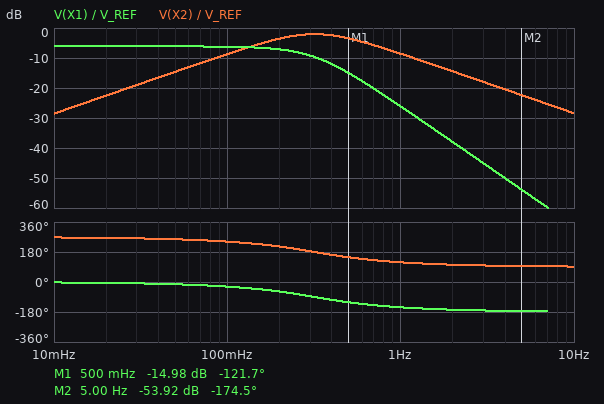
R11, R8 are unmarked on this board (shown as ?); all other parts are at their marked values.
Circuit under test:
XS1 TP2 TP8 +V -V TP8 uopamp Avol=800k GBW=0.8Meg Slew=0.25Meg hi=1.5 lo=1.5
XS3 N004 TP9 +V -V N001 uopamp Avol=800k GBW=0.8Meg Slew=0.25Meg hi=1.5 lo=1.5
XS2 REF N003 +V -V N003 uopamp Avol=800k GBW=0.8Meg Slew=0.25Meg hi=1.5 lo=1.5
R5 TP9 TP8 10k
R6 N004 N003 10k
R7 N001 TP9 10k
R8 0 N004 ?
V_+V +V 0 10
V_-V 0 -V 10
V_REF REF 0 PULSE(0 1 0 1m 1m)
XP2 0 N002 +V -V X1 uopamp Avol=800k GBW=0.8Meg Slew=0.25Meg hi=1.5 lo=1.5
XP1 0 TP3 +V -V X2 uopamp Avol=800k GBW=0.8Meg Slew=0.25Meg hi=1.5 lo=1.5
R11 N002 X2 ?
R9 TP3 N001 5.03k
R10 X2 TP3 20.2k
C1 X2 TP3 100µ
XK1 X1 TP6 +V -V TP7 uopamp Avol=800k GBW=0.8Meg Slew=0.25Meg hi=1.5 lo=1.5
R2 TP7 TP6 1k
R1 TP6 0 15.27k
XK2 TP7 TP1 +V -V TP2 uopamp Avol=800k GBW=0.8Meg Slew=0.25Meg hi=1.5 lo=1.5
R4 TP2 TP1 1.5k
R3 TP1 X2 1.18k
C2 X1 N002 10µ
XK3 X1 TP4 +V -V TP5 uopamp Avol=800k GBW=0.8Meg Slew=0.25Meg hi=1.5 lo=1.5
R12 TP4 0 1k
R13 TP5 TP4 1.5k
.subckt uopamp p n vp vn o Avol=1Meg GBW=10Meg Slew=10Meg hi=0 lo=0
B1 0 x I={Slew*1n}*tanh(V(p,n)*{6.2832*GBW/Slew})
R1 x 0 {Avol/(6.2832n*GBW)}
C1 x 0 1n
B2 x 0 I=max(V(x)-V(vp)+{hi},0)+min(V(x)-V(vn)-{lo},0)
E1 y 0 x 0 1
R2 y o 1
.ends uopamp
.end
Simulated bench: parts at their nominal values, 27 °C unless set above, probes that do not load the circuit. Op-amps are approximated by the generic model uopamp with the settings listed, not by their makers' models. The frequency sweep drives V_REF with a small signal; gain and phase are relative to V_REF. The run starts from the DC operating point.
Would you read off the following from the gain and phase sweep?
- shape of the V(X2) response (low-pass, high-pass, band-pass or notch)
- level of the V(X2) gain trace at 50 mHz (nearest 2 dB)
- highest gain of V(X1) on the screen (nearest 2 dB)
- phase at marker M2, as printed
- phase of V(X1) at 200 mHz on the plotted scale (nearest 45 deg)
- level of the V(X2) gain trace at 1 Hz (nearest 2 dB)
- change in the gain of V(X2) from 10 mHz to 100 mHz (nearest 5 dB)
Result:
band-pass
-14 dB
-6 dB
-174.5 deg
-45 deg
-8 dB
20 dB
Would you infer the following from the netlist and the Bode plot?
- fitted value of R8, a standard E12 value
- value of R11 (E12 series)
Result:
15 kΩ
120 kΩ
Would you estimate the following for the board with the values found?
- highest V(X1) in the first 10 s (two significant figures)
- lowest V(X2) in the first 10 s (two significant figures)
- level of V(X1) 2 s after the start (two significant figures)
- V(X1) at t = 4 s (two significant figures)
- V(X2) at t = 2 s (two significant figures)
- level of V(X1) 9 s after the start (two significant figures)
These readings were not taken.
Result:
510 mV
-520 mV
500 mV
500 mV
-44 mV
500 mV
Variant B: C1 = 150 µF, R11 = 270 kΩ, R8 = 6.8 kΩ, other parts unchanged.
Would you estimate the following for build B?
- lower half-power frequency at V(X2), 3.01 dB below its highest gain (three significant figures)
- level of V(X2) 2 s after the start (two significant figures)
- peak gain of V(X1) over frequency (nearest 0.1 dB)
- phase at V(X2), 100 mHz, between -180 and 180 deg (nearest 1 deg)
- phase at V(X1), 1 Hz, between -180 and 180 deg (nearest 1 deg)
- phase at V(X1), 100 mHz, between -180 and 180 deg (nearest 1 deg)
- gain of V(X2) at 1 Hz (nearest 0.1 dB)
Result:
75.9 mHz
-250 mV
-9.5 dB
-148 deg
-162 deg
-58 deg
-15.5 dB
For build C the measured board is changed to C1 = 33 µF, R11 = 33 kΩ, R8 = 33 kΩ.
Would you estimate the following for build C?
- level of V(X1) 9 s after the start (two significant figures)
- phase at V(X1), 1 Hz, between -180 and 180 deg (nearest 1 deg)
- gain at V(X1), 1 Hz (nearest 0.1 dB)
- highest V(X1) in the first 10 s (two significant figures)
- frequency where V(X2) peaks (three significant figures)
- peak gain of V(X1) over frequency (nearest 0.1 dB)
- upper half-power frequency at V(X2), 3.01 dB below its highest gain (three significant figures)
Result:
630 mV
-85 deg
-6.3 dB
670 mV
1.06 Hz
-3.9 dB
2.01 Hz
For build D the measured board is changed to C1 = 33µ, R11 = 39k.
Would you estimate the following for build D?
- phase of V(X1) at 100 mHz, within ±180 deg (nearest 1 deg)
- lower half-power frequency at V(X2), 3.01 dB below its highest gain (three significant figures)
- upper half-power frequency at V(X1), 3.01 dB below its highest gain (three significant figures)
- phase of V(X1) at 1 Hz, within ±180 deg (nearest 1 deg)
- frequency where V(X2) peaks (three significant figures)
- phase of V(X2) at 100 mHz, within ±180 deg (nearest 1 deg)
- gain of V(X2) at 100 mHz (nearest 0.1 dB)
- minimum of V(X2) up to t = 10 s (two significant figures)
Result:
-9 deg
487 mHz
916 mHz
-92 deg
973 mHz
-99 deg
-18.3 dB
-520 mV
